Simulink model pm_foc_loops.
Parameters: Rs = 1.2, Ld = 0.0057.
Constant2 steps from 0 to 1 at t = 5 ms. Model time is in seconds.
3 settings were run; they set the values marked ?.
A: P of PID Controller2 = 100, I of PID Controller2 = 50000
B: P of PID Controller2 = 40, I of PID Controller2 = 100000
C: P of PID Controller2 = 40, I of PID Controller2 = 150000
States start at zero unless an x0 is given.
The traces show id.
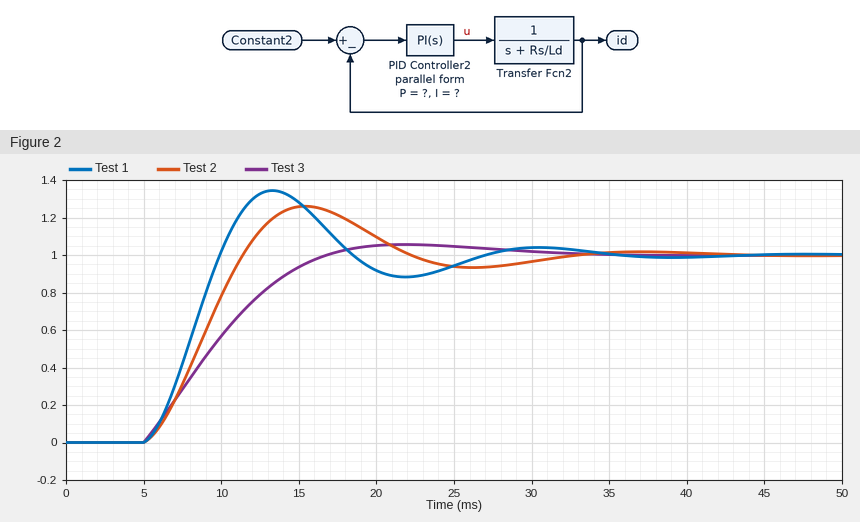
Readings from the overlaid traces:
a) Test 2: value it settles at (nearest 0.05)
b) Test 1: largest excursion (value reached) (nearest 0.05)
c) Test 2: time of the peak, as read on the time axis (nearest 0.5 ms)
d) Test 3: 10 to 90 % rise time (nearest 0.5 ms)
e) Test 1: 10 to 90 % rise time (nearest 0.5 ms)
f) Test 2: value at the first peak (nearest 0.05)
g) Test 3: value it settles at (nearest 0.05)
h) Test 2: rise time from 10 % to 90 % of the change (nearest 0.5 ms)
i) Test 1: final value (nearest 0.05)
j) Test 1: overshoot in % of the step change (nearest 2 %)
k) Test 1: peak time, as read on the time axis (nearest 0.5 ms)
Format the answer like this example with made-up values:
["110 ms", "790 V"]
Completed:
["1.00", "1.35", "15.5 ms", "8.5 ms", "3.5 ms", "1.25", "1.00", "4.5 ms", "1.00", "34 %", "13.5 ms"]
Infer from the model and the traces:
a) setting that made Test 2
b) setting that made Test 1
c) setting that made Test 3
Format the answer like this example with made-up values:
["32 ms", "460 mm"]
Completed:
["B", "C", "A"]
